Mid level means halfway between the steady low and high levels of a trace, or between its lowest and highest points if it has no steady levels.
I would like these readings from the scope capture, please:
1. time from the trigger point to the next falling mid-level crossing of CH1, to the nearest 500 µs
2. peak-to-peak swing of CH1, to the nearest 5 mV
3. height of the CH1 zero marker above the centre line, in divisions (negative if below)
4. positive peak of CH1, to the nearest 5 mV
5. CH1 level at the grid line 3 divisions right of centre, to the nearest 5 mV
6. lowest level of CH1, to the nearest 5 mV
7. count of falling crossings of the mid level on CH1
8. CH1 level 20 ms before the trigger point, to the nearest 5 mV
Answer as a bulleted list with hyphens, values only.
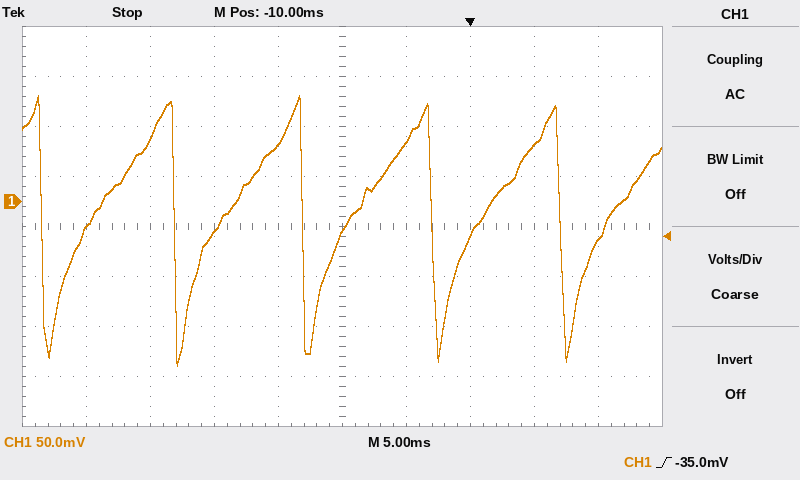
- 7.0 ms
- 270 mV
- +0.5 div
- 105 mV
- 55 mV
- -165 mV
- 5
- -30 mV
